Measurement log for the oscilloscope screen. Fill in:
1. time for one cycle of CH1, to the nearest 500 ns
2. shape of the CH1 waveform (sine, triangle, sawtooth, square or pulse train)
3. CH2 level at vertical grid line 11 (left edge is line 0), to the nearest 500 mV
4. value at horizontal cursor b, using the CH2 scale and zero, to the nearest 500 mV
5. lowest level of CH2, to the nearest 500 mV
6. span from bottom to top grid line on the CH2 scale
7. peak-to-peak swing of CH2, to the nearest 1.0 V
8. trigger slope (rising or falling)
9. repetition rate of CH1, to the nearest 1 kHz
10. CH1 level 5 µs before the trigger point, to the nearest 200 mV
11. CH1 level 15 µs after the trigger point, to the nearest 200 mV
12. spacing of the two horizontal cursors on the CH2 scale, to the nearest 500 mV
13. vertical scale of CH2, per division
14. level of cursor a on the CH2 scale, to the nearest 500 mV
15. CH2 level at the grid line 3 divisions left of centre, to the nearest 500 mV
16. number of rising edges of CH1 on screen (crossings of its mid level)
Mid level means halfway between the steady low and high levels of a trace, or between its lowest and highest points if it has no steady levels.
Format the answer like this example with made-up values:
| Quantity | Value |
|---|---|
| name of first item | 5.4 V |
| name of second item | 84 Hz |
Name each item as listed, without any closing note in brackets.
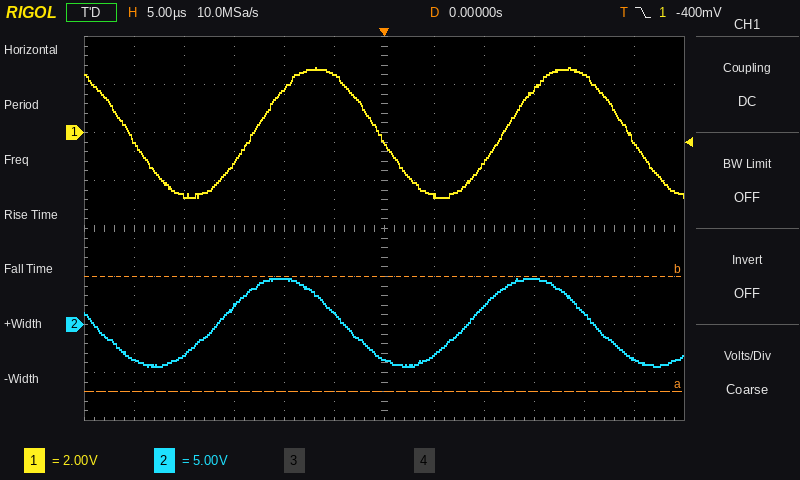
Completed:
| Quantity | Value |
|---|---|
| time for one cycle of CH1, to the nearest 500 ns | 25.0 µs |
| shape of the CH1 waveform | sine |
| CH2 level at vertical grid line 11 (left edge is line 0), to the nearest 500 mV | -3.5 V |
| value at horizontal cursor b, using the CH2 scale and zero, to the nearest 500 mV | 5.0 V |
| lowest level of CH2, to the nearest 500 mV | -4.5 V |
| span from bottom to top grid line on the CH2 scale | 40 V |
| peak-to-peak swing of CH2, to the nearest 1.0 V | 9.0 V |
| trigger slope | falling |
| repetition rate of CH1, to the nearest 1 kHz | 40 kHz |
| CH1 level 5 µs before the trigger point, to the nearest 200 mV | 2.4 V |
| CH1 level 15 µs after the trigger point, to the nearest 200 mV | 1.8 V |
| spacing of the two horizontal cursors on the CH2 scale, to the nearest 500 mV | 12.0 V |
| vertical scale of CH2, per division | 5 V |
| level of cursor a on the CH2 scale, to the nearest 500 mV | -7.0 V |
| CH2 level at the grid line 3 divisions left of centre, to the nearest 500 mV | 2.0 V |
| number of rising edges of CH1 on screen | 2 |
